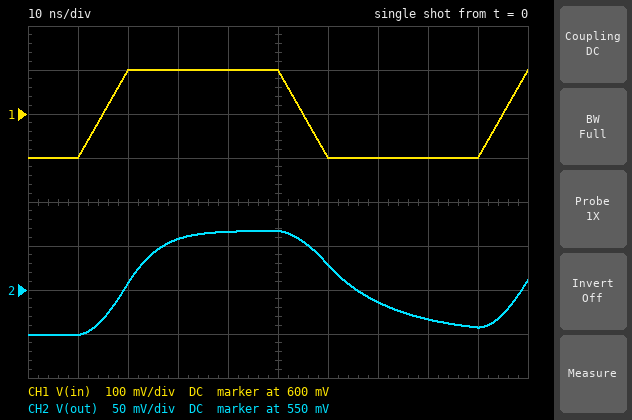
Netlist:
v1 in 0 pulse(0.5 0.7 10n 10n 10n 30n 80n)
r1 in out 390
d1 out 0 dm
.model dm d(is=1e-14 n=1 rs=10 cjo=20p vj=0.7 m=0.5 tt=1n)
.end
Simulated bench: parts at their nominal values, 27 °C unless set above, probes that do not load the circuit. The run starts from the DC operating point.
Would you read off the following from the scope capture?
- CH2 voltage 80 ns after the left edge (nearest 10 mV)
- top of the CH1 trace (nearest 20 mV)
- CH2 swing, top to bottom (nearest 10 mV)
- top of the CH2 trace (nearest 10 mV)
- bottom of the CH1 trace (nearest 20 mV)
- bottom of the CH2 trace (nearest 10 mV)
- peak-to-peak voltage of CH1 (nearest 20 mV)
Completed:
520 mV
700 mV
120 mV
620 mV
500 mV
500 mV
200 mV
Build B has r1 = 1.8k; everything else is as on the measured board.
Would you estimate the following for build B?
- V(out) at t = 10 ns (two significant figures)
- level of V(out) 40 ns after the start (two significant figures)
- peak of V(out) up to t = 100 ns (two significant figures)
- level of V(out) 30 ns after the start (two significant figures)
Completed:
500 mV
560 mV
570 mV
540 mV
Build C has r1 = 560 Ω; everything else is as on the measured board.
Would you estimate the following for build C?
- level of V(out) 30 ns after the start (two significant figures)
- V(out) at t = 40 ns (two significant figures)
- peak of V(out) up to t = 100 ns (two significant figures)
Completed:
590 mV
610 mV
610 mV
